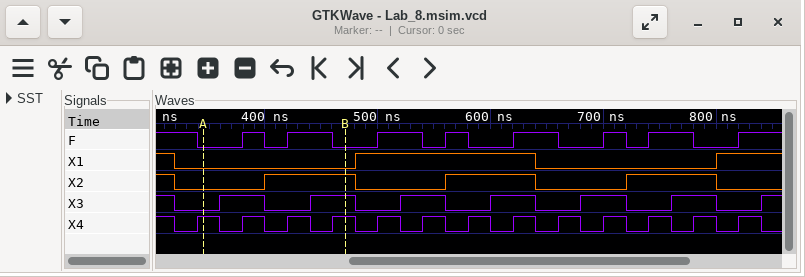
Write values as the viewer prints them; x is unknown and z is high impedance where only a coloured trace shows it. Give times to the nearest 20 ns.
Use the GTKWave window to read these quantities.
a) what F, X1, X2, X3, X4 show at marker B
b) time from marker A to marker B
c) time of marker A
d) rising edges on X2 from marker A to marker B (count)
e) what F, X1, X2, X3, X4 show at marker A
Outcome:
F=0, X1=0, X2=1, X3=1, X4=1
120 ns
340 ns
1
F=0, X1=0, X2=0, X3=0, X4=1
